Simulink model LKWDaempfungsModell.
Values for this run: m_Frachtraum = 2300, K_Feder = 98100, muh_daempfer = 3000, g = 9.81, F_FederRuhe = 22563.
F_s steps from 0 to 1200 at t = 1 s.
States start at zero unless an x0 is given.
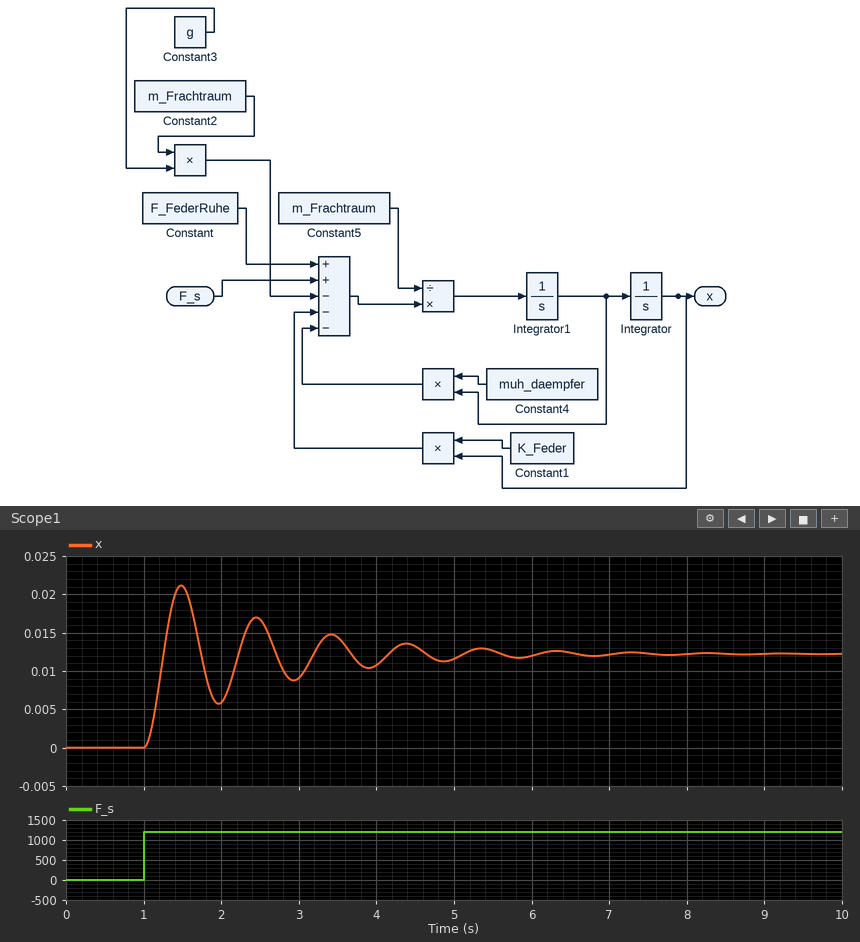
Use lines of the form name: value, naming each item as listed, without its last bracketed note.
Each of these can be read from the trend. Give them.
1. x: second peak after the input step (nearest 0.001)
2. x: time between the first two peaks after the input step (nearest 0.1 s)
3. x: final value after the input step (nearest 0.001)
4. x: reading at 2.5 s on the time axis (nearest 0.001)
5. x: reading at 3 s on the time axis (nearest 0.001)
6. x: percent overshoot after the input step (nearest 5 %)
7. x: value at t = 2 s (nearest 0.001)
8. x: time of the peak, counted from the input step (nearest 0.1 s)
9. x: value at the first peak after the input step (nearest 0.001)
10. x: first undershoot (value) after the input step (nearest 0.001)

x: second peak after the input step: 0.017
x: time between the first two peaks after the input step: 1.0 s
x: final value after the input step: 0.012
x: reading at 2.5 s on the time axis: 0.017
x: reading at 3 s on the time axis: 0.009
x: percent overshoot after the input step: 75 %
x: value at t = 2 s: 0.006
x: time of the peak, counted from the input step: 0.5 s
x: value at the first peak after the input step: 0.021
x: first undershoot (value) after the input step: 0.006
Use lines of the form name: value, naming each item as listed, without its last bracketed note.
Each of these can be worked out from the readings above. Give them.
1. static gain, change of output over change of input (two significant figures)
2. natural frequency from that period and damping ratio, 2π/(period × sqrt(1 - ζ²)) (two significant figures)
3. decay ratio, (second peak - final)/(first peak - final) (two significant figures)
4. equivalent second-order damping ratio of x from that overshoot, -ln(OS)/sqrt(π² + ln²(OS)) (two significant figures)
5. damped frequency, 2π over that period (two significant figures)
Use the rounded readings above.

static gain, change of output over change of input: 0.000010
natural frequency from that period and damping ratio, 2π/(period × sqrt(1 - ζ²)): 6.3 rad/s
decay ratio, (second peak - final)/(first peak - final): 0.56
equivalent second-order damping ratio of x from that overshoot, -ln(OS)/sqrt(π² + ln²(OS)): 0.091
damped frequency, 2π over that period: 6.3 rad/s
